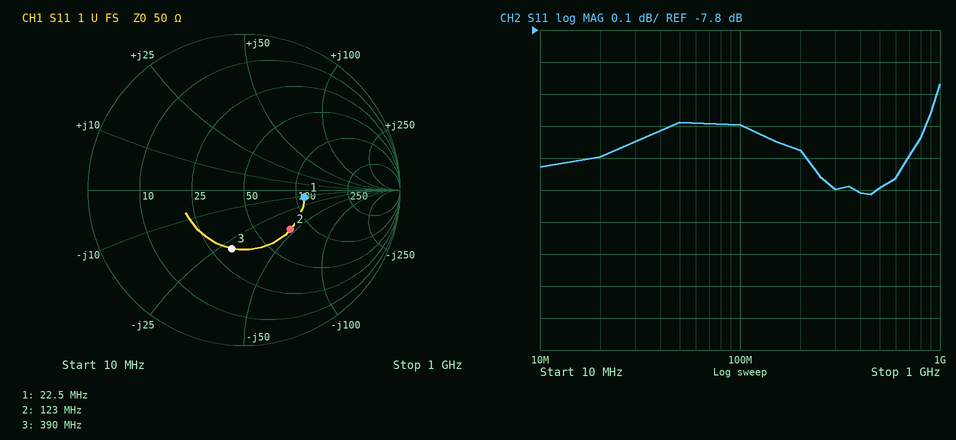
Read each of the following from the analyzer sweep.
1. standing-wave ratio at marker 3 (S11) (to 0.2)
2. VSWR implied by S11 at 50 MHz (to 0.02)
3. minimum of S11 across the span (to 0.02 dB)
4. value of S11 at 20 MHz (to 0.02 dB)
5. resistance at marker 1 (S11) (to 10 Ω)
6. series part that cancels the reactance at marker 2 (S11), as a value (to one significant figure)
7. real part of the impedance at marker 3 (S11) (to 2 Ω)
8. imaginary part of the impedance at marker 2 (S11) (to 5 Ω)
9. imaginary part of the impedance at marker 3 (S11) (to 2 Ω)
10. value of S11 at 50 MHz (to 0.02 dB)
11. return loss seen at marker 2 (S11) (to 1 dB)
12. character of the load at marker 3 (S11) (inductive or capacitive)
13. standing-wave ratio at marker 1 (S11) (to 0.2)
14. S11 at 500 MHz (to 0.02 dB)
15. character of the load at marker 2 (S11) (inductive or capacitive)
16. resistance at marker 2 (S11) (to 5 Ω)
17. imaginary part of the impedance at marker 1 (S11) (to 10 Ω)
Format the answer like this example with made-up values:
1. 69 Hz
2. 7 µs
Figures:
1. 2.2
2. 2.30
3. -8.32 dB
4. -8.20 dB
5. 110 Ω
6. 60 nH
7. 32 Ω
8. -45 Ω
9. -28 Ω
10. -8.08 dB
11. 8 dB
12. capacitive
13. 2.2
14. -8.30 dB
15. capacitive
16. 75 Ω
17. -10 Ω
